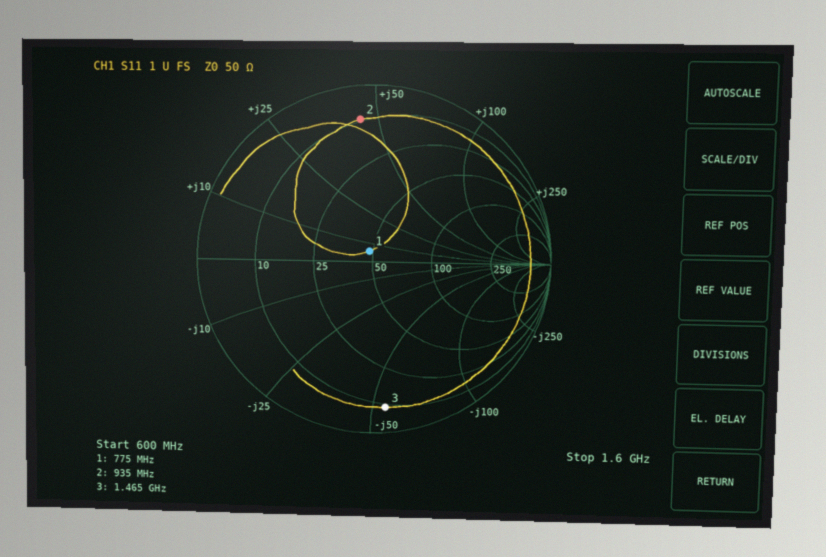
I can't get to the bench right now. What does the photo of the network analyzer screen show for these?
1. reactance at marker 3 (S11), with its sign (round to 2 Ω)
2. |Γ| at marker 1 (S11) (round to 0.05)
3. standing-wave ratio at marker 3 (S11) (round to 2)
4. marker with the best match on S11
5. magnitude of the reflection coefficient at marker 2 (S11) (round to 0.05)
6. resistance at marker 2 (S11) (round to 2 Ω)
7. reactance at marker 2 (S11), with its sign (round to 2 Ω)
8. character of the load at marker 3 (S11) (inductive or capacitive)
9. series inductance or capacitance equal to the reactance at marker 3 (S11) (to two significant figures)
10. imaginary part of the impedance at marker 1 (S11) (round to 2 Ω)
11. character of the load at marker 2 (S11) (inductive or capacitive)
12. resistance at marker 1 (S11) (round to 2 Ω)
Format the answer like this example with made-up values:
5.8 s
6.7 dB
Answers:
-54 Ω
0.05
12
marker 1
0.80
10 Ω
+44 Ω
capacitive
2.0 pF
+6 Ω
inductive
48 Ω
